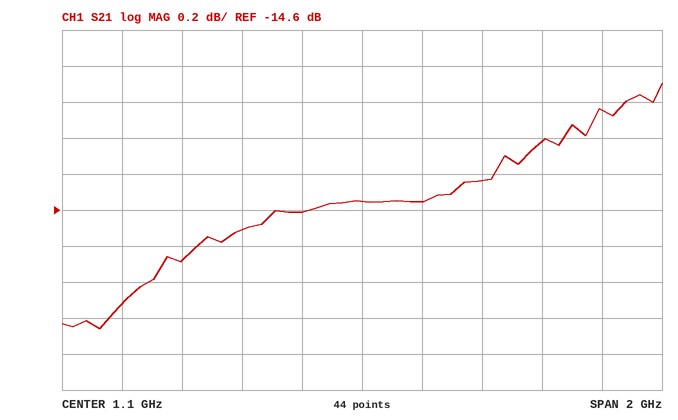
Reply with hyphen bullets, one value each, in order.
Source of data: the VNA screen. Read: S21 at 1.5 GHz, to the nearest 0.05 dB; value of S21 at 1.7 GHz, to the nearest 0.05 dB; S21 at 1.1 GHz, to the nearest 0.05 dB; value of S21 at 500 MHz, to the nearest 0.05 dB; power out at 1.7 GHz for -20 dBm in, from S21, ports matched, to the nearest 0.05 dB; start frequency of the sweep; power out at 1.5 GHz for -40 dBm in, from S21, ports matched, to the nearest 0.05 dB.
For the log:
- -14.45 dB
- -14.20 dB
- -14.55 dB
- -14.90 dB
- -34.20 dBm
- 100 MHz
- -54.45 dBm
